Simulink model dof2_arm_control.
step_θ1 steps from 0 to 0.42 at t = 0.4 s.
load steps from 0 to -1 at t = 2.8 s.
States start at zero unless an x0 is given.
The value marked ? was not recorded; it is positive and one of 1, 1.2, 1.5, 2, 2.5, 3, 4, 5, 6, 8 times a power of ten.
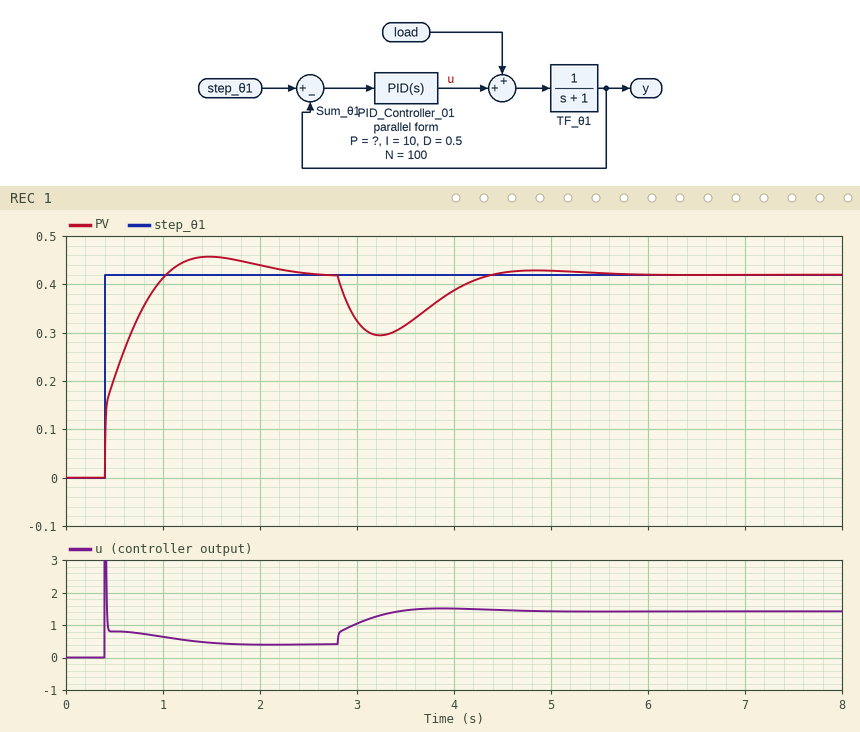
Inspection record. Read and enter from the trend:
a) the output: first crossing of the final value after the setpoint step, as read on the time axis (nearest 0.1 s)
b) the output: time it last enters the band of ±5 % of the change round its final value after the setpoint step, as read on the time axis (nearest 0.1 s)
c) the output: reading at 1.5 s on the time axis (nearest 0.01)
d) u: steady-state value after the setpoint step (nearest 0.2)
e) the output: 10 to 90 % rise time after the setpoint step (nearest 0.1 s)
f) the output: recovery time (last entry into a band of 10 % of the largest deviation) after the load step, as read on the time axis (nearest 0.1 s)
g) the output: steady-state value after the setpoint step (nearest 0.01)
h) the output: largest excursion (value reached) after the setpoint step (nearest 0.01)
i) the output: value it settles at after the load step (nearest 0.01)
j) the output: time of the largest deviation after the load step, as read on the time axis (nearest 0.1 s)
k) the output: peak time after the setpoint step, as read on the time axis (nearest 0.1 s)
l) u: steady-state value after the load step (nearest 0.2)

1.0 s
2.0 s
0.46
0.4
0.5 s
4.2 s
0.42
0.46
0.42
3.2 s
1.5 s
1.4
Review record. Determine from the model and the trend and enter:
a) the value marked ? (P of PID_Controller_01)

4
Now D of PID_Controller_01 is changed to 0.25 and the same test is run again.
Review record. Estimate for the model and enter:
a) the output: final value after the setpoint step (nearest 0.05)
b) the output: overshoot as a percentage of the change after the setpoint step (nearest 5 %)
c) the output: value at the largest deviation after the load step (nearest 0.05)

0.40
10 %
0.30
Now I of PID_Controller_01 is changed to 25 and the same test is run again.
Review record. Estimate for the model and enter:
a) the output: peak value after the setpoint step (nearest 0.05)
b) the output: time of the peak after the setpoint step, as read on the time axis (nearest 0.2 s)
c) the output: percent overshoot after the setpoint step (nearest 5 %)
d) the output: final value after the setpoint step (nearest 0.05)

0.50
1.0 s
20 %
0.40
